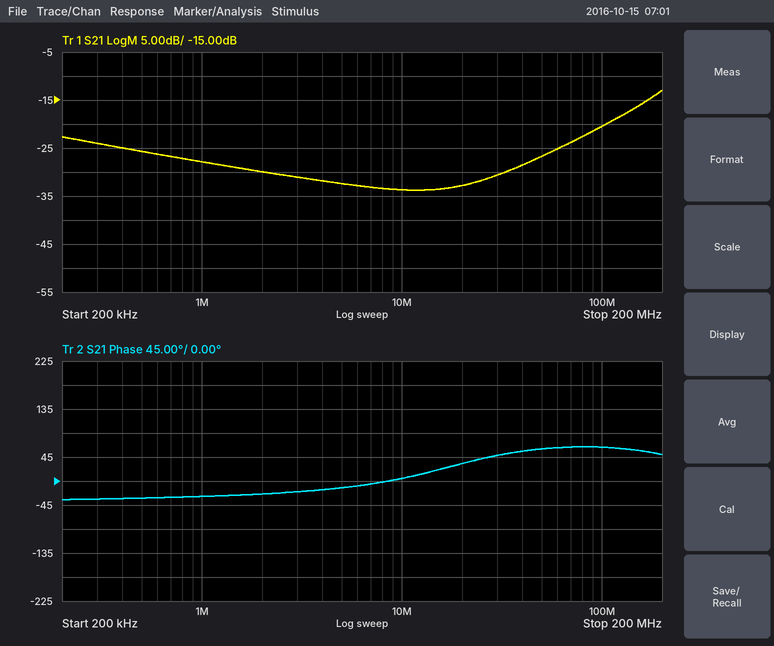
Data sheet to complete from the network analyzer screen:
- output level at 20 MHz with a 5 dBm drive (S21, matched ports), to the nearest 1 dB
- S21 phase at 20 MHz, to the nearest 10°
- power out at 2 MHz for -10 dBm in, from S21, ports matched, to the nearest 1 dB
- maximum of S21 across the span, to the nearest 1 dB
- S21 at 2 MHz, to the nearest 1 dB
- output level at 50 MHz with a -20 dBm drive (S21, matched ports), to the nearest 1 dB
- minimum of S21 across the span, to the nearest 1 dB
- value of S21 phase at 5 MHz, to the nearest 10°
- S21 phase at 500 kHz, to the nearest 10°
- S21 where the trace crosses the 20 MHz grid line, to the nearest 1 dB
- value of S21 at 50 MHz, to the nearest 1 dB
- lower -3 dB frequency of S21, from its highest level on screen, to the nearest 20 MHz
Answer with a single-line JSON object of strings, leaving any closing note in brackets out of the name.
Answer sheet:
{"output level at 20 MHz with a 5 dBm drive (S21, matched ports), to the nearest 1 dB": "-28 dBm", "S21 phase at 20 MHz, to the nearest 10°": "30°", "power out at 2 MHz for -10 dBm in, from S21, ports matched, to the nearest 1 dB": "-40 dBm", "maximum of S21 across the span, to the nearest 1 dB": "-13 dB", "S21 at 2 MHz, to the nearest 1 dB": "-30 dB", "output level at 50 MHz with a -20 dBm drive (S21, matched ports), to the nearest 1 dB": "-47 dBm", "minimum of S21 across the span, to the nearest 1 dB": "-34 dB", "value of S21 phase at 5 MHz, to the nearest 10°": "-10°", "S21 phase at 500 kHz, to the nearest 10°": "-30°", "S21 where the trace crosses the 20 MHz grid line, to the nearest 1 dB": "-33 dB", "value of S21 at 50 MHz, to the nearest 1 dB": "-27 dB", "lower -3 dB frequency of S21, from its highest level on screen, to the nearest 20 MHz": "160 MHz"}
